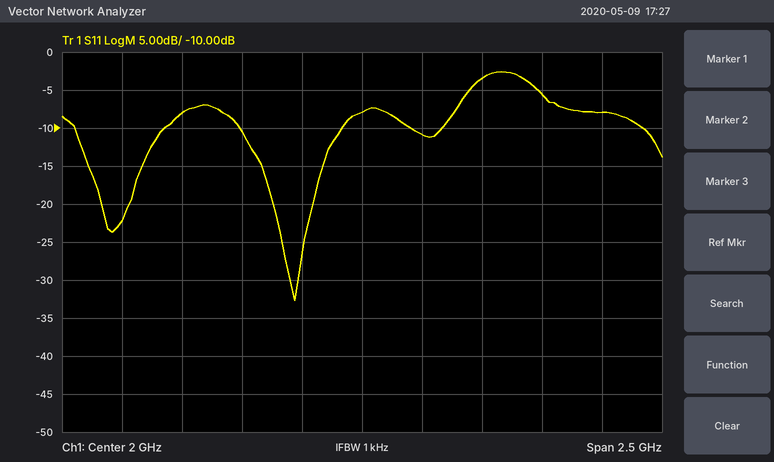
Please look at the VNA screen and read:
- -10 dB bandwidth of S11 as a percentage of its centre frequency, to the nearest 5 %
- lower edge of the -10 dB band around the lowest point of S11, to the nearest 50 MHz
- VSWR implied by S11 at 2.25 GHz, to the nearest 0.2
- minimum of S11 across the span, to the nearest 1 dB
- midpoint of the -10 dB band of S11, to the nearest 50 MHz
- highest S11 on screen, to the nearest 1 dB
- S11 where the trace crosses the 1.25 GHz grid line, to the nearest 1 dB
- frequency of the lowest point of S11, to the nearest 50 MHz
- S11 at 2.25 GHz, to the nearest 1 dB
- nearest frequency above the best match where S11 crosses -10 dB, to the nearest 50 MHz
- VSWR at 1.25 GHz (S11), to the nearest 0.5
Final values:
25 %
1.50 GHz
1.8
-33 dB
1.70 GHz
-3 dB
-8 dB
1.70 GHz
-11 dB
1.90 GHz
2.5
